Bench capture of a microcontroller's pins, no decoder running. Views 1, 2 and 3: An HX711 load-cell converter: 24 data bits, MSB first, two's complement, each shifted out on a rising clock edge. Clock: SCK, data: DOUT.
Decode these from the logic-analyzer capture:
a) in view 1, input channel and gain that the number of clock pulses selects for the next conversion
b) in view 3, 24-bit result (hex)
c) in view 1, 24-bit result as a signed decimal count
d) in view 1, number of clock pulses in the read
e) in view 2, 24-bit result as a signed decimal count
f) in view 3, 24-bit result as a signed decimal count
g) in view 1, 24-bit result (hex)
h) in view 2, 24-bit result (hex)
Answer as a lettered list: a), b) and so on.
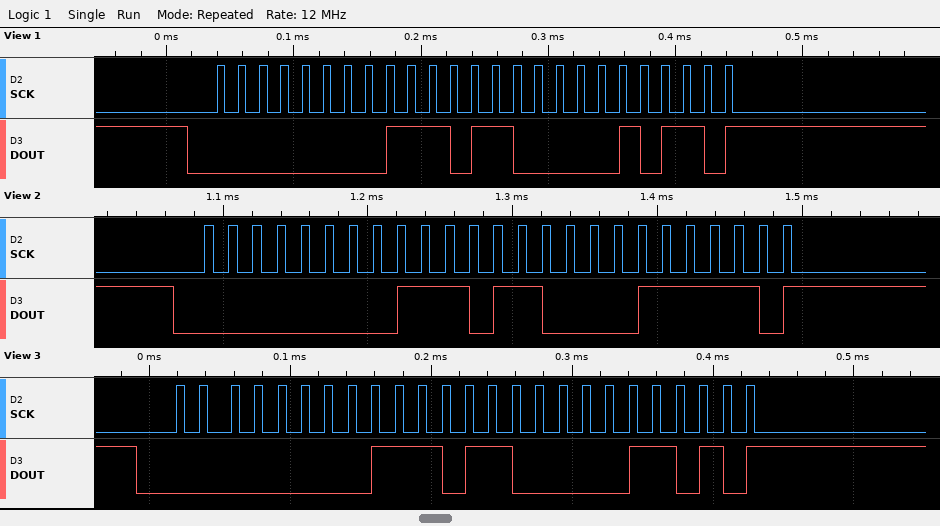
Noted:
a) channel A, gain 128
b) 0x00EC1A
c) 60438
d) 25
e) 60478
f) 60442
g) 0x00EC16
h) 0x00EC3E
